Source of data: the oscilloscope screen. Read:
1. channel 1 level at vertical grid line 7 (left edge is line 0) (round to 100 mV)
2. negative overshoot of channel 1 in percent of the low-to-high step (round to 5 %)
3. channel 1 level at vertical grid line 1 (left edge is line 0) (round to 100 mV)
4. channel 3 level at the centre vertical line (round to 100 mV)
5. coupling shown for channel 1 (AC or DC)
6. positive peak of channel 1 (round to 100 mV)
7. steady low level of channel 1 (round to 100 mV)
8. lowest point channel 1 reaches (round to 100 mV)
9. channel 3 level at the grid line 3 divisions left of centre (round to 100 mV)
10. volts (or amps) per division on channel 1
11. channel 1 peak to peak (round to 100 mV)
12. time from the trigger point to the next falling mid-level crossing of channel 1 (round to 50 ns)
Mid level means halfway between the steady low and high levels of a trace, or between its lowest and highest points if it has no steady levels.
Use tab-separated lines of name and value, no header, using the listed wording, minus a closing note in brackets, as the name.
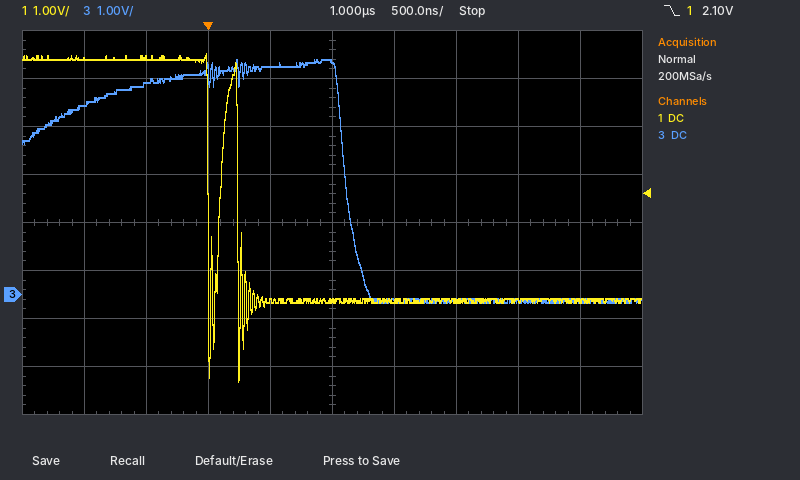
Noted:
channel 1 level at vertical grid line 7 (left edge is line 0)	-100 mV
negative overshoot of channel 1 in percent of the low-to-high step	35 %
channel 1 level at vertical grid line 1 (left edge is line 0)	4.9 V
channel 3 level at the centre vertical line	4.8 V
coupling shown for channel 1	DC
positive peak of channel 1	5.0 V
steady low level of channel 1	-100 mV
lowest point channel 1 reaches	-1.8 V
channel 3 level at the grid line 3 divisions left of centre	4.4 V
volts (or amps) per division on channel 1	1 V
channel 1 peak to peak	6.8 V
time from the trigger point to the next falling mid-level crossing of channel 1	250 ns
